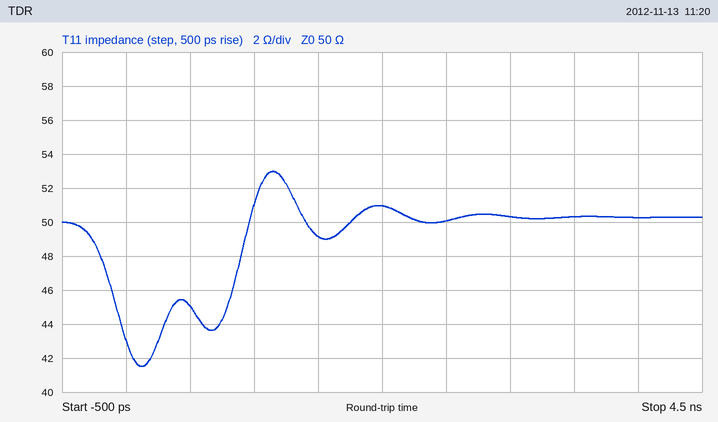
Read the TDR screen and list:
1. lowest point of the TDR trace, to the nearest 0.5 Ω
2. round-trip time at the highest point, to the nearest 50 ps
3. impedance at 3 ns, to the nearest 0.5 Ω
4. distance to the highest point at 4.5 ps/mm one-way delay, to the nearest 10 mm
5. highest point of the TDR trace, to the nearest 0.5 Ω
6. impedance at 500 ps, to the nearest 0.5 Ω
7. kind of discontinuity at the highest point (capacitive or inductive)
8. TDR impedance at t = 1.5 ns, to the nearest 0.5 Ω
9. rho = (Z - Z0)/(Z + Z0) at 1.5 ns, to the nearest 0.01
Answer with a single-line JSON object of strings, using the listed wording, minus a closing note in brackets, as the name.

{"lowest point of the TDR trace, to the nearest 0.5 Ω": "41.5 Ω", "round-trip time at the highest point, to the nearest 50 ps": "1.15 ns", "impedance at 3 ns, to the nearest 0.5 Ω": "50.5 Ω", "distance to the highest point at 4.5 ps/mm one-way delay, to the nearest 10 mm": "130 mm", "highest point of the TDR trace, to the nearest 0.5 Ω": "53.0 Ω", "impedance at 500 ps, to the nearest 0.5 Ω": "45.0 Ω", "kind of discontinuity at the highest point": "inductive", "TDR impedance at t = 1.5 ns, to the nearest 0.5 Ω": "49.0 Ω", "rho = (Z - Z0)/(Z + Z0) at 1.5 ns, to the nearest 0.01": "-0.01"}
